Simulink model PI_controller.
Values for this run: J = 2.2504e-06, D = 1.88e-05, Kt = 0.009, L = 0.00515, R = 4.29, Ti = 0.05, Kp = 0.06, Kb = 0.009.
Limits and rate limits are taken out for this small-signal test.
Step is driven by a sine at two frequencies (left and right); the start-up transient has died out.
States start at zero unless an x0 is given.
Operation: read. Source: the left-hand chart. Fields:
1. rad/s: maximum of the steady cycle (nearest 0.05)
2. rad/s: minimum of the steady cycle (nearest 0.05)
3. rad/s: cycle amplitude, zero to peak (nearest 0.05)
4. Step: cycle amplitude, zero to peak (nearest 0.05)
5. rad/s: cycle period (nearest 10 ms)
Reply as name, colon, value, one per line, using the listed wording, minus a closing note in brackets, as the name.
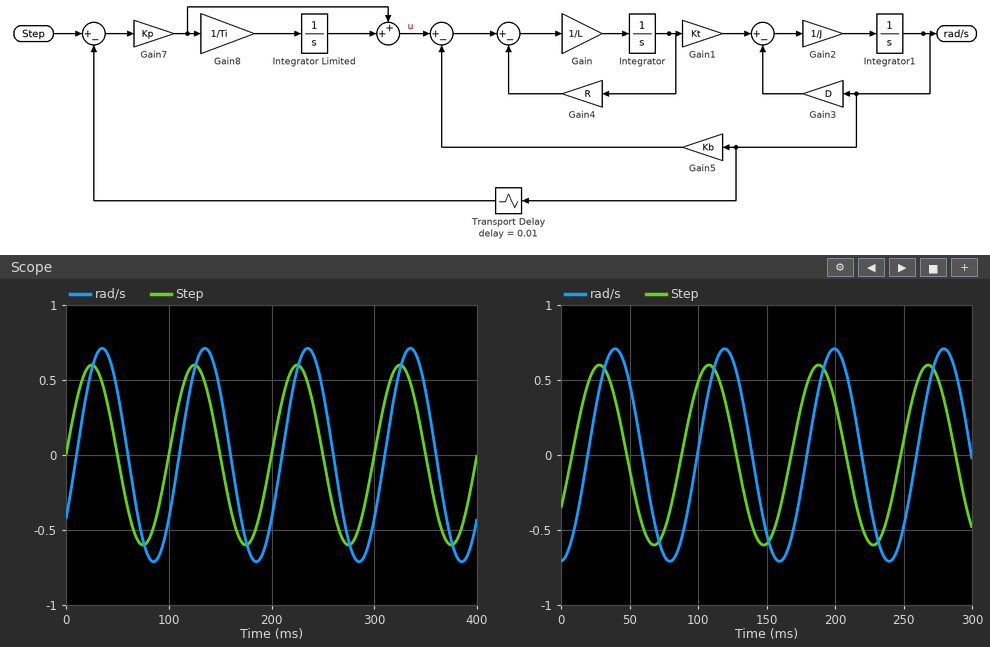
rad/s: maximum of the steady cycle: 0.70
rad/s: minimum of the steady cycle: -0.70
rad/s: cycle amplitude, zero to peak: 0.70
Step: cycle amplitude, zero to peak: 0.60
rad/s: cycle period: 100 ms
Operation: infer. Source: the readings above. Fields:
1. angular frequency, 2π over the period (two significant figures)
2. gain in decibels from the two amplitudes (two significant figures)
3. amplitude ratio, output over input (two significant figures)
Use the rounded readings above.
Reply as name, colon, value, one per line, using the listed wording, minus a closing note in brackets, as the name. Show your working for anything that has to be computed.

angular frequency, 2π over the period: 2π / 100 = 0.063 rad/ms
gain in decibels from the two amplitudes: 20 log10(0.7 / 0.6) = 1.3 dB
amplitude ratio, output over input: 0.7 / 0.6 = 1.2
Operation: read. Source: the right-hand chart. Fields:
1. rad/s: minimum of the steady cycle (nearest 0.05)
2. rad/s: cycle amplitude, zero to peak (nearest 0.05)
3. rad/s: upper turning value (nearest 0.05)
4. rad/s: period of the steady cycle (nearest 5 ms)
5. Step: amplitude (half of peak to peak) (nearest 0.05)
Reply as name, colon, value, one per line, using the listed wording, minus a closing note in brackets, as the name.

rad/s: minimum of the steady cycle: -0.70
rad/s: cycle amplitude, zero to peak: 0.70
rad/s: upper turning value: 0.70
rad/s: period of the steady cycle: 80 ms
Step: amplitude (half of peak to peak): 0.60
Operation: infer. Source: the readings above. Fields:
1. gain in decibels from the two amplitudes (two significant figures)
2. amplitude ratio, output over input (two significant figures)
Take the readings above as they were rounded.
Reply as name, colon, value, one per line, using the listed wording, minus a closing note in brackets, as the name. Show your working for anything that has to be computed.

gain in decibels from the two amplitudes: 20 log10(0.7 / 0.6) = 1.3 dB
amplitude ratio, output over input: 0.7 / 0.6 = 1.2
